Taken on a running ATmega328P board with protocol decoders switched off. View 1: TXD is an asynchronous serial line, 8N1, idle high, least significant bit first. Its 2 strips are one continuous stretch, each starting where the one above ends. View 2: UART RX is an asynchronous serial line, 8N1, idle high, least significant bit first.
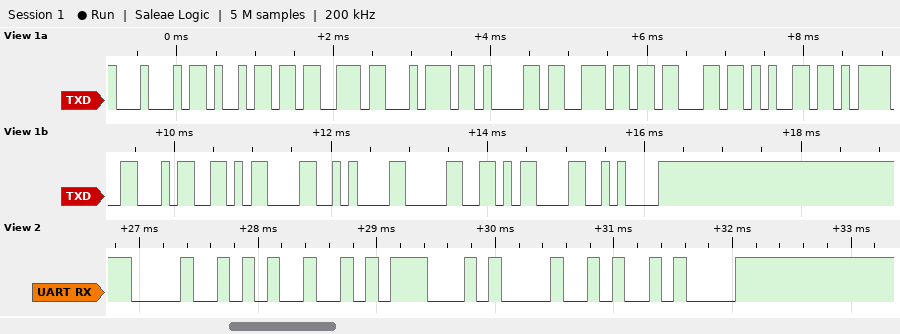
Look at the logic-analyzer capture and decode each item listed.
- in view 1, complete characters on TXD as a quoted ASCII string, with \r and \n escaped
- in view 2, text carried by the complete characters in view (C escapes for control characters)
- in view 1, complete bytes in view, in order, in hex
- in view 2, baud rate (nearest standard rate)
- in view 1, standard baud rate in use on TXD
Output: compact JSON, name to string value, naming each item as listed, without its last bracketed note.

{"in view 1, complete characters on TXD as a quoted ASCII string, with \\r and \\n escaped": "\"Distance=4\\r\\n0\\r\\n\"", "in view 2, text carried by the complete characters in view": "\"HIGH\\n\"", "in view 1, complete bytes in view, in order, in hex": "0x44 0x69 0x73 0x74 0x61 0x6E 0x63 0x65 0x3D 0x34 0x0D 0x0A 0x30 0x0D 0x0A", "in view 2, baud rate": "9600 baud", "in view 1, standard baud rate in use on TXD": "9600 baud"}
